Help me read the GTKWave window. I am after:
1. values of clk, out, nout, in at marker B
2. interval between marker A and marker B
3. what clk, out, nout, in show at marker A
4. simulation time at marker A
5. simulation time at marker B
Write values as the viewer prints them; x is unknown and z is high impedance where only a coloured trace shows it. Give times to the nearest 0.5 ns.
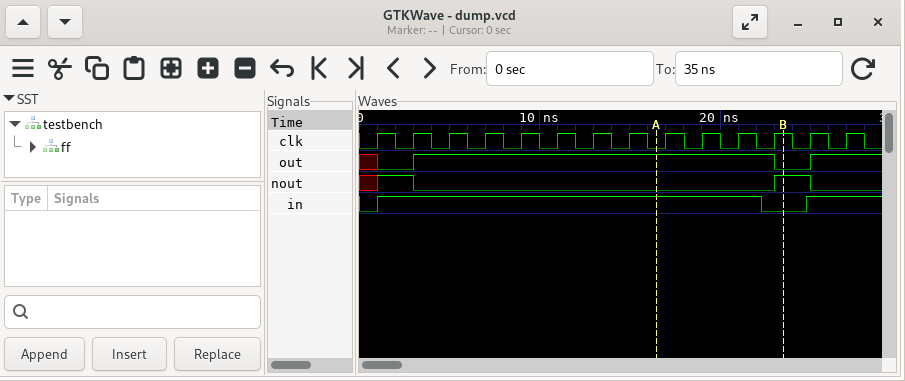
clk=1, out=0, nout=1, in=0
7 ns
clk=0, out=1, nout=0, in=1
16.5 ns
23.5 ns
